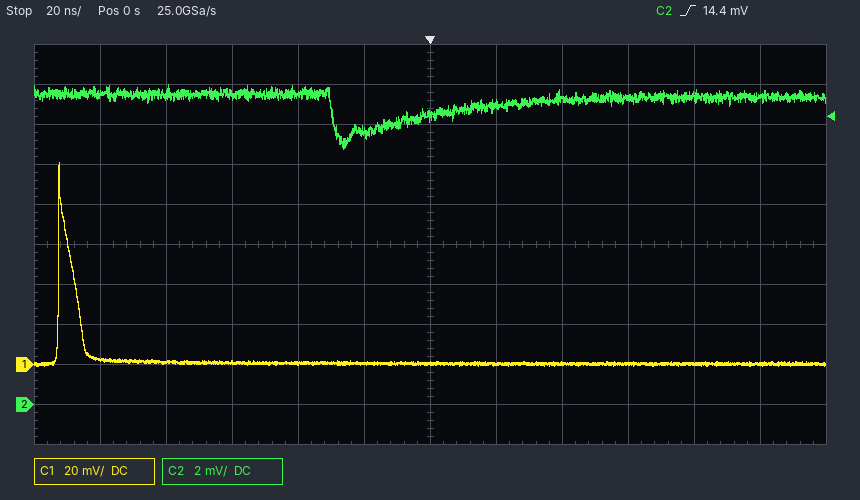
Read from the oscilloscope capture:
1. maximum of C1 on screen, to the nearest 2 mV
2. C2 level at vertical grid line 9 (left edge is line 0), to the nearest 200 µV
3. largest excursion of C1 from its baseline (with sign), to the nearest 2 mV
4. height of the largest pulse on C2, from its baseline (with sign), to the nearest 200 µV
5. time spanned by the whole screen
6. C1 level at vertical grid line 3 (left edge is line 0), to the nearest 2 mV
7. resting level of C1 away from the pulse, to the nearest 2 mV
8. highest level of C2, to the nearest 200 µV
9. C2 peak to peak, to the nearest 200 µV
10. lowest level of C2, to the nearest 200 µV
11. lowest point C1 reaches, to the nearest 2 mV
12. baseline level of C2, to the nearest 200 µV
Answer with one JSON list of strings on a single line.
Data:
["100 mV", "15.4 mV", "+100 mV", "-2.6 mV", "240 ns", "2 mV", "0 mV", "16.0 mV", "3.2 mV", "12.8 mV", "0 mV", "15.4 mV"]
